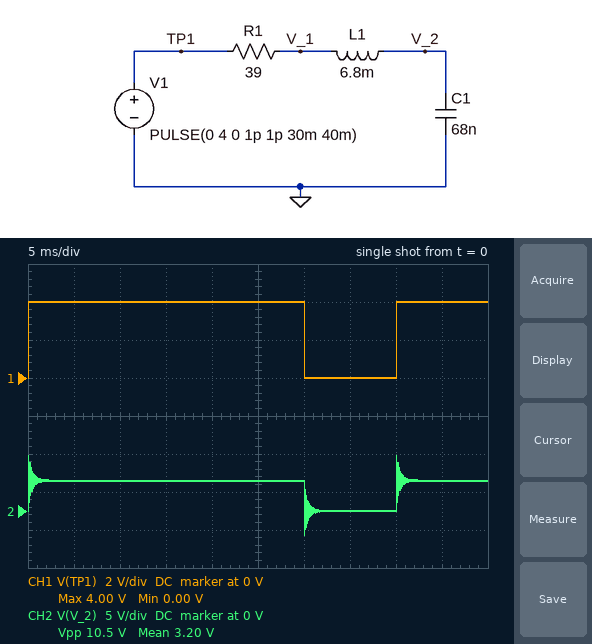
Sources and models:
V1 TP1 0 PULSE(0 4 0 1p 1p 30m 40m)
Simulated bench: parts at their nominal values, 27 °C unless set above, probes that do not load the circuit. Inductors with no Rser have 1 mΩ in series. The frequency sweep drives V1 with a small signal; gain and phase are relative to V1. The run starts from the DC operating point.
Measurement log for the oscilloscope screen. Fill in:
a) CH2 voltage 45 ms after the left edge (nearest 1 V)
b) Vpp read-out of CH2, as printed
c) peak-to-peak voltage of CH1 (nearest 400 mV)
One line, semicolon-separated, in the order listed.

4 V; 10.5 V; 4.0 V
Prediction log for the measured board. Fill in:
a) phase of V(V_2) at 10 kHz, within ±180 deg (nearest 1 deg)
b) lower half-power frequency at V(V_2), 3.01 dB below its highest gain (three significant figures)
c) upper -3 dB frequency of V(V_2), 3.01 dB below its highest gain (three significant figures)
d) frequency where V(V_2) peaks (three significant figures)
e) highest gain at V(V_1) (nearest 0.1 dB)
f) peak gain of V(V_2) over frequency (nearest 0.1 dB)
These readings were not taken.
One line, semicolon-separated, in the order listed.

-169 deg; 6.90 kHz; 7.82 kHz; 7.37 kHz; 0 dB; 18.2 dB
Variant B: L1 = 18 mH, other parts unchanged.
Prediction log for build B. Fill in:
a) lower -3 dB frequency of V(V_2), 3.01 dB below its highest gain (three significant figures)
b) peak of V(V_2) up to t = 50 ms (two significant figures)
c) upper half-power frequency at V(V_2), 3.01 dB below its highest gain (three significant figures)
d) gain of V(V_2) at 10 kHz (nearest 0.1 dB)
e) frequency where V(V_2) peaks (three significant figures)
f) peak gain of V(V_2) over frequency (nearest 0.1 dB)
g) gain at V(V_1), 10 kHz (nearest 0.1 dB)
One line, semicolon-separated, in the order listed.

4.37 kHz; 7.5 V; 4.71 kHz; -11.7 dB; 4.54 kHz; 22.4 dB; 0 dB
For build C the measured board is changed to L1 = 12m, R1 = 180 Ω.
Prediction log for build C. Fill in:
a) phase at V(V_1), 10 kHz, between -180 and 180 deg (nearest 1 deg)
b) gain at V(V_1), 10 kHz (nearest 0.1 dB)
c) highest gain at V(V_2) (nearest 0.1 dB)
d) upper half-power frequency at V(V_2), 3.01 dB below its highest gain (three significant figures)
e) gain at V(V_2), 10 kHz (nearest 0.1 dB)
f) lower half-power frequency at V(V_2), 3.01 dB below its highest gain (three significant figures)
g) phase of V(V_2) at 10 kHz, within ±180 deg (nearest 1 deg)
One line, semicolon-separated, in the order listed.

19 deg; -0.5 dB; 7.6 dB; 6.42 kHz; -7.4 dB; 3.90 kHz; -161 deg
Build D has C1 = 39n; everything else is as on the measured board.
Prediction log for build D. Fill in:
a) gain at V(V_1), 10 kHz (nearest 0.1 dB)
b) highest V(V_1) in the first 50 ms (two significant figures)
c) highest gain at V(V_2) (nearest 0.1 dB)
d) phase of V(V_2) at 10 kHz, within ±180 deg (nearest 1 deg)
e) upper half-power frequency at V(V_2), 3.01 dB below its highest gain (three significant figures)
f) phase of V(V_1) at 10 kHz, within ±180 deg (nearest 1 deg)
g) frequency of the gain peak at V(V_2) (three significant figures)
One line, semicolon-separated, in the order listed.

-7.1 dB; 4.3 V; 20.6 dB; -116 deg; 10.2 kHz; 64 deg; 9.75 kHz
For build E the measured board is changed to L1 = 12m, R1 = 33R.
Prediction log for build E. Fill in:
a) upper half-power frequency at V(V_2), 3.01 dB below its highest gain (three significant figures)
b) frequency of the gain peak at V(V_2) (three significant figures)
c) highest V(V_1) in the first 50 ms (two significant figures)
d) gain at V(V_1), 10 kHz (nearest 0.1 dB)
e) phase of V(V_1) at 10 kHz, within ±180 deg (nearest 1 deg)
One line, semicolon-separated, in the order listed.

5.78 kHz; 5.56 kHz; 4.3 V; 0 dB; 4 deg
